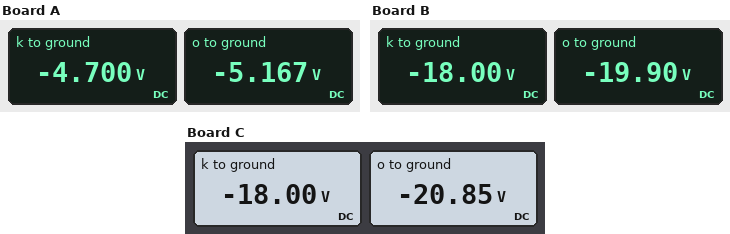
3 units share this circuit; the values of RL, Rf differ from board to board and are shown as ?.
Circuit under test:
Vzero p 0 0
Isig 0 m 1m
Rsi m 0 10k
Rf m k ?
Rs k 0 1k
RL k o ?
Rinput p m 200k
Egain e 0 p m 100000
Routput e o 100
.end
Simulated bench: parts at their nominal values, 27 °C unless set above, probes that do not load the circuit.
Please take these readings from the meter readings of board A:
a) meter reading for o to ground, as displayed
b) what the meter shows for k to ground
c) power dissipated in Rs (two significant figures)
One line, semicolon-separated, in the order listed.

-5.167 V; -4.700 V; 22 mW
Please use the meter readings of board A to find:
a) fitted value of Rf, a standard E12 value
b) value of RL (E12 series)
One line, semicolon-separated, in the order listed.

4.7 kΩ; 82 Ω
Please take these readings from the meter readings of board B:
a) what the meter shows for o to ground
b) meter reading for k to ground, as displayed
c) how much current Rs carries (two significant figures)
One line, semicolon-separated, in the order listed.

-19.90 V; -18.00 V; 18 mA
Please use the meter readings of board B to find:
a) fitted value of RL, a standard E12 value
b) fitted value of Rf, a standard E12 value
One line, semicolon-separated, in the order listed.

100 Ω; 18 kΩ
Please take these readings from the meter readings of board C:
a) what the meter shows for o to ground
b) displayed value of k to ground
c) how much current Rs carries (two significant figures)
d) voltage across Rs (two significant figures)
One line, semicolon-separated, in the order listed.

-20.85 V; -18.00 V; 18 mA; 18 V
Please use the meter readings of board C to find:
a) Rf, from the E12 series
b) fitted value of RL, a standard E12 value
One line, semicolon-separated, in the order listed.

18 kΩ; 150 Ω
